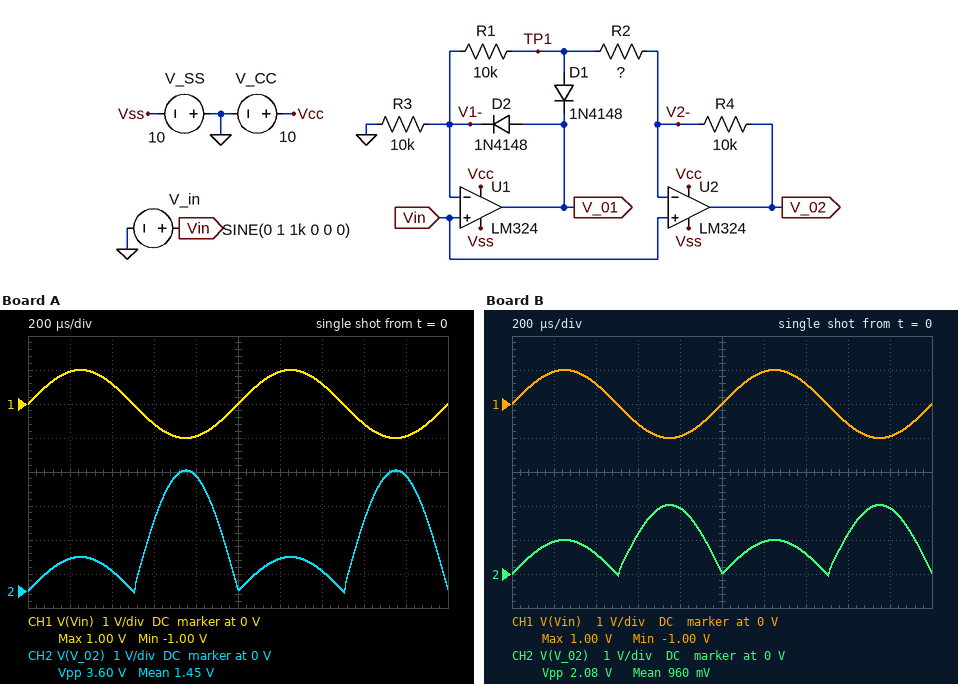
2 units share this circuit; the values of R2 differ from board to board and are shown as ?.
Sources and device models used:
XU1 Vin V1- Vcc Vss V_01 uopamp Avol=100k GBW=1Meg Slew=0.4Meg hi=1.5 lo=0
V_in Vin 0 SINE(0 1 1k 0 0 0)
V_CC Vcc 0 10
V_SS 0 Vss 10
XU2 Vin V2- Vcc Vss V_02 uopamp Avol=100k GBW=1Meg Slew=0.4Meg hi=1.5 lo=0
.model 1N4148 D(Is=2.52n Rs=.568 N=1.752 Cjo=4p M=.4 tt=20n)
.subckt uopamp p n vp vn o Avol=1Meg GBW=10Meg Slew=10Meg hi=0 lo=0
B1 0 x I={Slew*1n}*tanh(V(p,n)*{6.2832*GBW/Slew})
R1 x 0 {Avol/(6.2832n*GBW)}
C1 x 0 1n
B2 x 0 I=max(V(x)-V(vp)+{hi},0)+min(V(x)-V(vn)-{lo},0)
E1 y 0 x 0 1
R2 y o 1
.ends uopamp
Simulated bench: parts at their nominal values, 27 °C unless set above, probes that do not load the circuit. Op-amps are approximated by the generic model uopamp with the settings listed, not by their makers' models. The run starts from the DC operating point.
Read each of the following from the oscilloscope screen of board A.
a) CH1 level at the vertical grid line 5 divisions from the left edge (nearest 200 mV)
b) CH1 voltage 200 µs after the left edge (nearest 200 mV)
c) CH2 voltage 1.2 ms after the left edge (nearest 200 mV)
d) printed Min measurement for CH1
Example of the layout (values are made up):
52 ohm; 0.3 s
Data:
0 V; 1.0 V; 1.0 V; -1.00 V
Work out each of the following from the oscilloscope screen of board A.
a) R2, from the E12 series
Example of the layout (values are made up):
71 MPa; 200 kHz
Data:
2.2 kΩ
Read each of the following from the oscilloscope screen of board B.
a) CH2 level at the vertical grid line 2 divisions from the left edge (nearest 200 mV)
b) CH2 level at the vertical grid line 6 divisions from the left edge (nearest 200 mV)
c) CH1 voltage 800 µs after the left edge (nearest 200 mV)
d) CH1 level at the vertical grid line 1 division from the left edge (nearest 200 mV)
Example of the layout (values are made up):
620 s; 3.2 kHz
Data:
600 mV; 1.0 V; -1.0 V; 1.0 V
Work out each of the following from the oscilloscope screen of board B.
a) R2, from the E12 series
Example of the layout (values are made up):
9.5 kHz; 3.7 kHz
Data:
3.3 kΩ
